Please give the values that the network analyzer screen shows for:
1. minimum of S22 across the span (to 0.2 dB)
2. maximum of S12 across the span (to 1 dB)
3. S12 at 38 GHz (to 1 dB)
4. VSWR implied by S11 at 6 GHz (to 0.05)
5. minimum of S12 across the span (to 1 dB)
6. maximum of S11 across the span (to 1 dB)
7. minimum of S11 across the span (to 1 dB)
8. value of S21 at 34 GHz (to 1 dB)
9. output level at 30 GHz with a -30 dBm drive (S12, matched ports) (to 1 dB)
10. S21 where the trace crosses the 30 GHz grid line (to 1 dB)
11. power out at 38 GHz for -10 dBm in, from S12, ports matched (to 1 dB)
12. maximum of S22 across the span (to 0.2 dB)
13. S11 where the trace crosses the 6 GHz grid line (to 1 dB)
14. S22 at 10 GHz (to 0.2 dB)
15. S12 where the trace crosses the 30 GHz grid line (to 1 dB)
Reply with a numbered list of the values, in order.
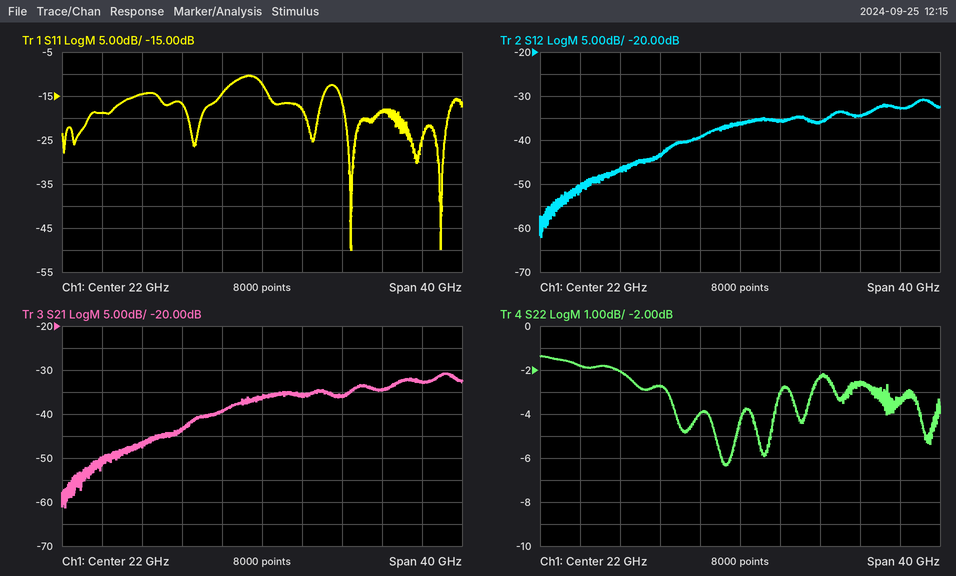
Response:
1. -6.4 dB
2. -31 dB
3. -33 dB
4. 1.25
5. -62 dB
6. -10 dB
7. -50 dB
8. -34 dB
9. -66 dBm
10. -36 dB
11. -43 dBm
12. -1.4 dB
13. -19 dB
14. -2.0 dB
15. -36 dB
